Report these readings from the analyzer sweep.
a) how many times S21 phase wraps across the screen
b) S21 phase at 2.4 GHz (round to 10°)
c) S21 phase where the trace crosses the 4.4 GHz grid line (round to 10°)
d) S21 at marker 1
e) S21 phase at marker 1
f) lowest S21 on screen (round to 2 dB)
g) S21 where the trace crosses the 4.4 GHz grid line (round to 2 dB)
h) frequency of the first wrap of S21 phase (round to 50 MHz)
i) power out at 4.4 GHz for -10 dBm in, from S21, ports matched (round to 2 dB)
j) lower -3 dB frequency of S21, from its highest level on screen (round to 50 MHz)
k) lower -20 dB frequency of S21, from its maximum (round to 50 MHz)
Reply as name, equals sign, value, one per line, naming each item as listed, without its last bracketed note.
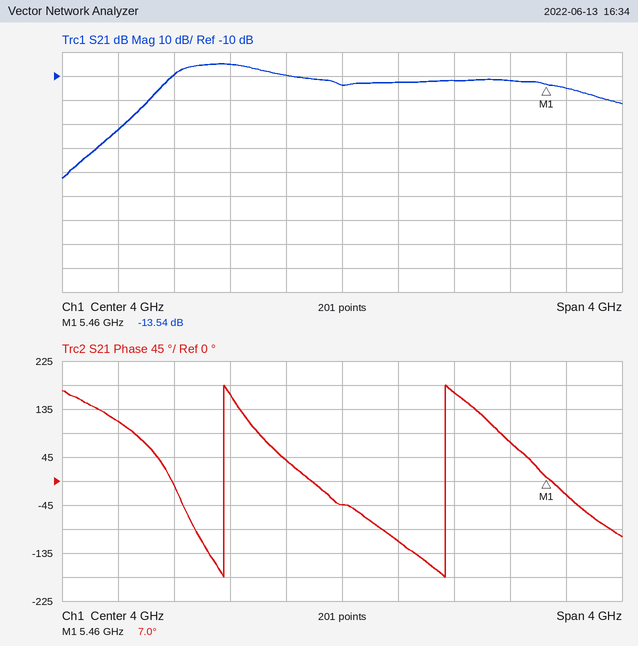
how many times S21 phase wraps across the screen = 2
S21 phase at 2.4 GHz = 110°
S21 phase where the trace crosses the 4.4 GHz grid line = -110°
S21 at marker 1 = -13.54 dB
S21 phase at marker 1 = 7.0°
lowest S21 on screen = -52 dB
S21 where the trace crosses the 4.4 GHz grid line = -12 dB
frequency of the first wrap of S21 phase = 3.15 GHz
power out at 4.4 GHz for -10 dBm in, from S21, ports matched = -22 dBm
lower -3 dB frequency of S21, from its highest level on screen = 2.85 GHz
lower -20 dB frequency of S21, from its maximum = 2.55 GHz
